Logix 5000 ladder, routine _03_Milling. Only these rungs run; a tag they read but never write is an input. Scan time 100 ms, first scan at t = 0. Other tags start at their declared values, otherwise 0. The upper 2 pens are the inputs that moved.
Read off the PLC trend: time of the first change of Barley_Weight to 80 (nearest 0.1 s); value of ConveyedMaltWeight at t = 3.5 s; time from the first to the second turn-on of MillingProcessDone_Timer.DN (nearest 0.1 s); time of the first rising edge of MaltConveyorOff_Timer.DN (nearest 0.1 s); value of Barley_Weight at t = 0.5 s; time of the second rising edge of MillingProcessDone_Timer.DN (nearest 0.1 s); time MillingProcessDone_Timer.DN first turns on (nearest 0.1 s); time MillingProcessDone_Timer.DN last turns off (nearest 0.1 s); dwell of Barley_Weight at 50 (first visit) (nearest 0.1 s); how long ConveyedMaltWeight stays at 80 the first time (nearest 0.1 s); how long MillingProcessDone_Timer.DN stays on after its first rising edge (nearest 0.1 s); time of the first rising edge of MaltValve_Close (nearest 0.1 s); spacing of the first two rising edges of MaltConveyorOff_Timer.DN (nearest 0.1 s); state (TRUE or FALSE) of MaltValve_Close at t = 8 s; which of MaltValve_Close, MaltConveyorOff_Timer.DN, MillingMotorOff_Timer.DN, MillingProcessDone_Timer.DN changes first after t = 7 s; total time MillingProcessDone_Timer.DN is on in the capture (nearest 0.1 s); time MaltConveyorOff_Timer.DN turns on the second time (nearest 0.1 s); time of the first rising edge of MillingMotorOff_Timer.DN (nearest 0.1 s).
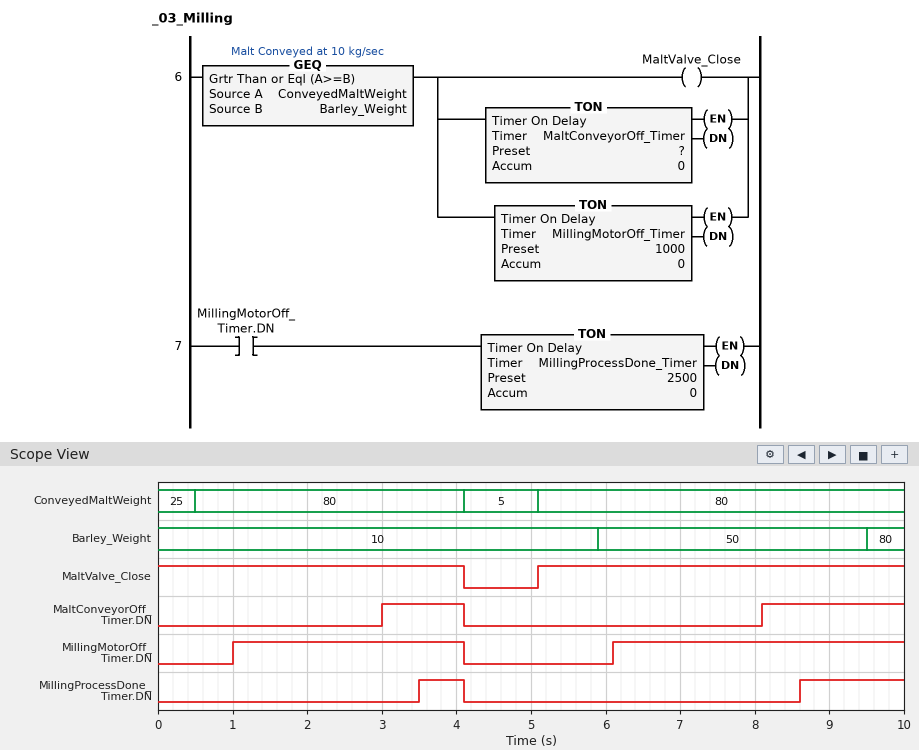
9.5 s
80
5.1 s
3.0 s
10
8.6 s
3.5 s
4.1 s
3.6 s
3.6 s
0.6 s
5.1 s
5.1 s
TRUE
MaltConveyorOff_Timer.DN
2.0 s
8.1 s
1.0 s
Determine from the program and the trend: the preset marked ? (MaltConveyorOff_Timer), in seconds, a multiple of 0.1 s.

3.0 s
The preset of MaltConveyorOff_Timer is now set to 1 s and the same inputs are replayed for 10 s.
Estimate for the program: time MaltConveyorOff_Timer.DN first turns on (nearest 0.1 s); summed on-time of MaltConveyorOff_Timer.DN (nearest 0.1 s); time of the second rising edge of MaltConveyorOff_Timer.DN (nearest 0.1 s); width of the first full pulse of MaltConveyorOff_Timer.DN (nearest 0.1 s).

1.0 s
7.0 s
6.1 s
3.1 s
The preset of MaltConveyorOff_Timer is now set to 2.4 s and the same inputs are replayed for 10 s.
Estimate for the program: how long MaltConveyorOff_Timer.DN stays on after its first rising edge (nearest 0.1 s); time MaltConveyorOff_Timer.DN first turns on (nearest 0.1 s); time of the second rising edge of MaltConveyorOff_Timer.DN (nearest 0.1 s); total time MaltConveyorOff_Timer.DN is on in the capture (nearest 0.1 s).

1.7 s
2.4 s
7.5 s
4.2 s
